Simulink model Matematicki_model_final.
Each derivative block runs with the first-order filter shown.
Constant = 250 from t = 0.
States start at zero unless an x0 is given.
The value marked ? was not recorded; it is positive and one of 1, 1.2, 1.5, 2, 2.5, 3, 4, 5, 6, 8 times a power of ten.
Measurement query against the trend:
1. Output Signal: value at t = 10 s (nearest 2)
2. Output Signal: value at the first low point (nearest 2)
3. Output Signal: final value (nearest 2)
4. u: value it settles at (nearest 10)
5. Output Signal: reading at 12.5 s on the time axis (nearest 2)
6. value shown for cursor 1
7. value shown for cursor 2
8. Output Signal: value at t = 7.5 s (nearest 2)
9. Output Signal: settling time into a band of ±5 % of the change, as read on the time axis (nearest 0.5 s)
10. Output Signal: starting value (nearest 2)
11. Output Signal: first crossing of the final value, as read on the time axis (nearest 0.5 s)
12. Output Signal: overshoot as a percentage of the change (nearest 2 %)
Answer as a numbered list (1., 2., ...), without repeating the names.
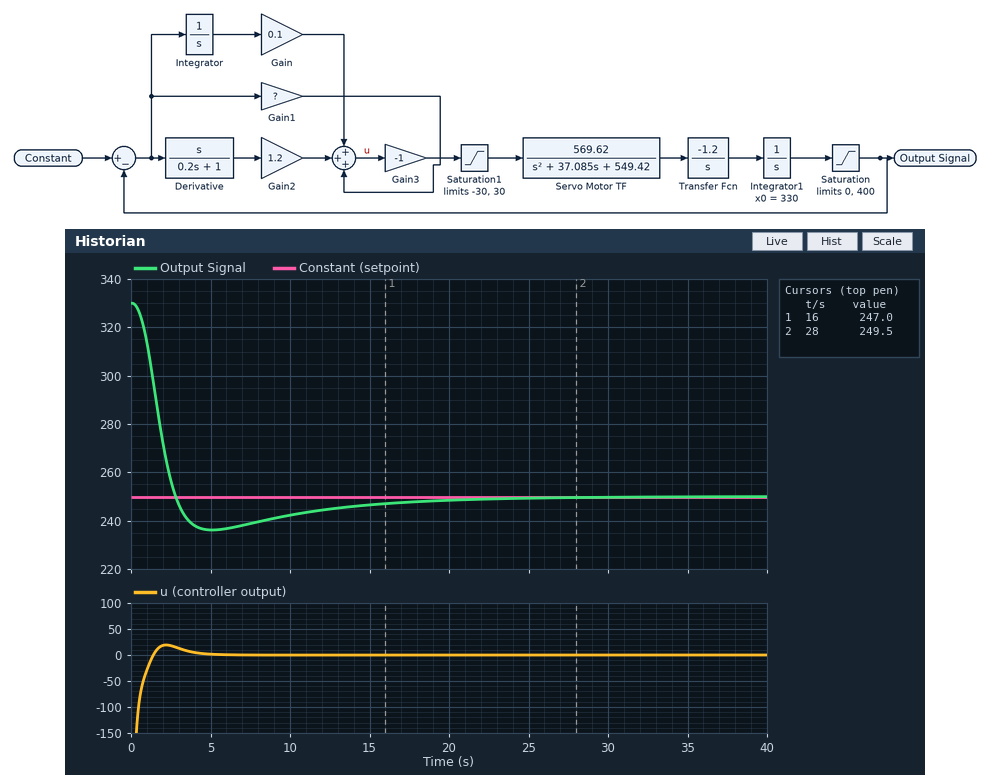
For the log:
1. 242
2. 236
3. 250
4. 0
5. 244
6. 247.0
7. 249.5
8. 238
9. 14.0 s
10. 330
11. 3.0 s
12. 18 %
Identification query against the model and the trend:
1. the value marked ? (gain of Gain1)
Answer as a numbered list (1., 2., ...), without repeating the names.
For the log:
1. 0.8
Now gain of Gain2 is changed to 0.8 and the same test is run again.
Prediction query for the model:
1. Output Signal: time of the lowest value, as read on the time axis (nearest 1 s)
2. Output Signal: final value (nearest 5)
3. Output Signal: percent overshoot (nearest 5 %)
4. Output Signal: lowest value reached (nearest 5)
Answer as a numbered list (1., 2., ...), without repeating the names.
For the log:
1. 4 s
2. 250
3. 35 %
4. 225
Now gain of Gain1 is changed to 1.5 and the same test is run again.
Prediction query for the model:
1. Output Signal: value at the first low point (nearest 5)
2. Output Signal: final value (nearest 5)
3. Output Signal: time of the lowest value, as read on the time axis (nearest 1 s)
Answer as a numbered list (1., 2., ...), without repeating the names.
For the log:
1. 230
2. 250
3. 3 s
